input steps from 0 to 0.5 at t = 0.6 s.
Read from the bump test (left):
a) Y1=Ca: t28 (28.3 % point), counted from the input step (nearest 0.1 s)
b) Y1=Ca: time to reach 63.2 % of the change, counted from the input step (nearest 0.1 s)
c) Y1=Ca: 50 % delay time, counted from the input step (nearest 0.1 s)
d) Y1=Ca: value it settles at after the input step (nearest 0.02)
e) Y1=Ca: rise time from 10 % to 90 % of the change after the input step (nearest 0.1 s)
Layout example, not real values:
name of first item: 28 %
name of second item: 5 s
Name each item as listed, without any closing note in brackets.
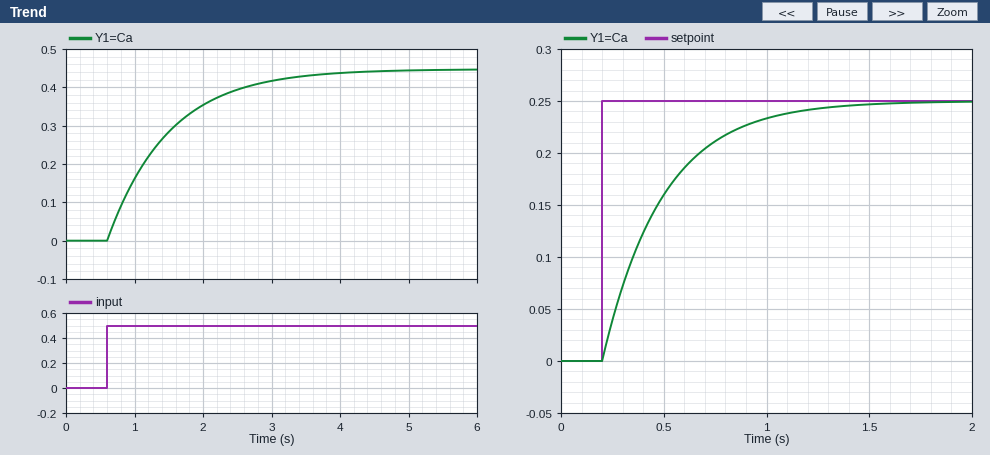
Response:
Y1=Ca: t28 (28.3 % point), counted from the input step: 0.3 s
Y1=Ca: time to reach 63.2 % of the change, counted from the input step: 0.9 s
Y1=Ca: 50 % delay time, counted from the input step: 0.6 s
Y1=Ca: value it settles at after the input step: 0.44
Y1=Ca: rise time from 10 % to 90 % of the change after the input step: 2.0 s
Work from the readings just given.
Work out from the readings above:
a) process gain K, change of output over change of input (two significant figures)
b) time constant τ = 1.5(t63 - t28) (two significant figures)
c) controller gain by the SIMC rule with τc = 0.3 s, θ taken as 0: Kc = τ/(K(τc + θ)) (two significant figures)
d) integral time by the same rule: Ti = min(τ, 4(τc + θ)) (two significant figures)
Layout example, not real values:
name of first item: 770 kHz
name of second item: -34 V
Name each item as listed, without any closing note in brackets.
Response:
process gain K, change of output over change of input: 0.88
time constant τ = 1.5(t63 - t28): 0.90 s
controller gain by the SIMC rule with τc = 0.3 s, θ taken as 0: Kc = τ/(K(τc + θ)): 3.4
integral time by the same rule: Ti = min(τ, 4(τc + θ)): 0.90 s
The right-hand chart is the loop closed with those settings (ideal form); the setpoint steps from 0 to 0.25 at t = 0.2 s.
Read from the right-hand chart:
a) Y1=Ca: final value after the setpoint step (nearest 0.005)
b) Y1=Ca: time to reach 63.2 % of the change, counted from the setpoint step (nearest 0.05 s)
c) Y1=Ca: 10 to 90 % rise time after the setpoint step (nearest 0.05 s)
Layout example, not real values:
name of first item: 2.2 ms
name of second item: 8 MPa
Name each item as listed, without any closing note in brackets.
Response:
Y1=Ca: final value after the setpoint step: 0.250
Y1=Ca: time to reach 63.2 % of the change, counted from the setpoint step: 0.30 s
Y1=Ca: 10 to 90 % rise time after the setpoint step: 0.65 s
